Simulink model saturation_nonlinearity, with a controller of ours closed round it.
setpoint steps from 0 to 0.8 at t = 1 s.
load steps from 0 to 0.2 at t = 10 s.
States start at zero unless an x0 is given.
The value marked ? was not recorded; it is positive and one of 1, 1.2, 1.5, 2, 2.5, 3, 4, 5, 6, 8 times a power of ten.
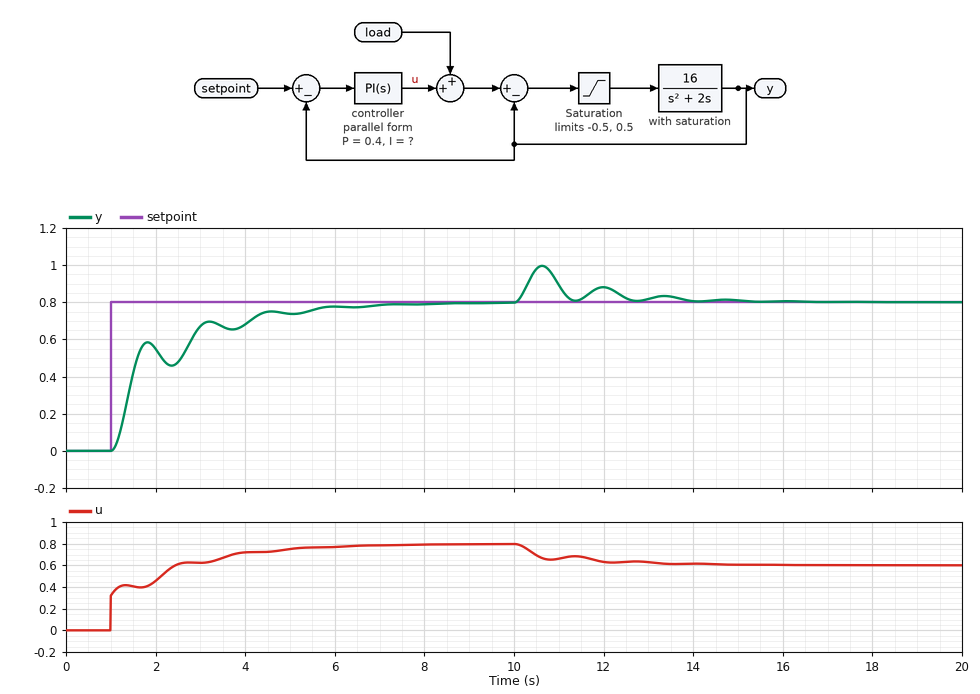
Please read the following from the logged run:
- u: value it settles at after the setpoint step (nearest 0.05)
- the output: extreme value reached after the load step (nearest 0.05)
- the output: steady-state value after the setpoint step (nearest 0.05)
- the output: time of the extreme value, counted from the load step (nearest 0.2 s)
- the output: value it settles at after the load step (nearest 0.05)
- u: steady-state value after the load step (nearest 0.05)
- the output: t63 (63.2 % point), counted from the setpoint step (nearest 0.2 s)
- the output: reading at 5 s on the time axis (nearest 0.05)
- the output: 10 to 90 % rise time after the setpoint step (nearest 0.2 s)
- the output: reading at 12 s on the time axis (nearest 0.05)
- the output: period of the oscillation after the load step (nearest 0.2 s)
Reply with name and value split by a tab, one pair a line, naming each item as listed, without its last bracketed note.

u: value it settles at after the setpoint step	0.80
the output: extreme value reached after the load step	1.00
the output: steady-state value after the setpoint step	0.80
the output: time of the extreme value, counted from the load step	0.6 s
the output: value it settles at after the load step	0.80
u: steady-state value after the load step	0.60
the output: t63 (63.2 % point), counted from the setpoint step	0.6 s
the output: reading at 5 s on the time axis	0.75
the output: 10 to 90 % rise time after the setpoint step	3.0 s
the output: reading at 12 s on the time axis	0.90
the output: period of the oscillation after the load step	1.4 s
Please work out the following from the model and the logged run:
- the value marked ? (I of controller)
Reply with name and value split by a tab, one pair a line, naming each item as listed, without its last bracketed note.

the value marked ?	0.8
